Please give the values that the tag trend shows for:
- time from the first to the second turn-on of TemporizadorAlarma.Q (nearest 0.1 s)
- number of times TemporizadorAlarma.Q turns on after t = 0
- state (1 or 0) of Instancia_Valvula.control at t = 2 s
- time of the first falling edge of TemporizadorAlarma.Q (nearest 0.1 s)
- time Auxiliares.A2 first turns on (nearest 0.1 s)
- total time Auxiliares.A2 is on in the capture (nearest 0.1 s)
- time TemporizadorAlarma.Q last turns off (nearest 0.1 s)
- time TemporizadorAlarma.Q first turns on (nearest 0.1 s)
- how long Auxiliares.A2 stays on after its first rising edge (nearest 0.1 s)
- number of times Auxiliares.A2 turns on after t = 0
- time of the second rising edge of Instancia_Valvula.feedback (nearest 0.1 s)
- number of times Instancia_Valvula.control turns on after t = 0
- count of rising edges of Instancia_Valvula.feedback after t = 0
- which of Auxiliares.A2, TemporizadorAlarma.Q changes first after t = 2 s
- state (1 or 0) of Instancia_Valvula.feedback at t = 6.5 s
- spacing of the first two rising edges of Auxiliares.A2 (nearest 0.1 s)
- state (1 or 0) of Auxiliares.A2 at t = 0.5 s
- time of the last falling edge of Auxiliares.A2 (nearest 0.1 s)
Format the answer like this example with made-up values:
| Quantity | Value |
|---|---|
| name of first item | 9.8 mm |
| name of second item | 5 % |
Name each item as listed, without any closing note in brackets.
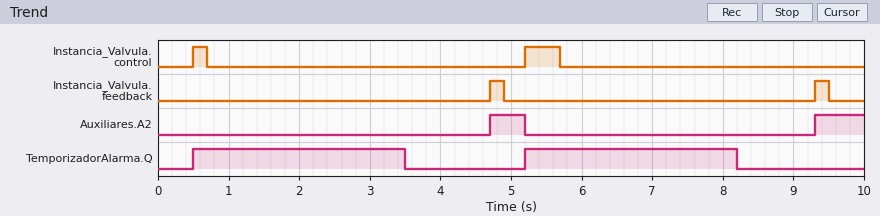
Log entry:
| Quantity | Value |
|---|---|
| time from the first to the second turn-on of TemporizadorAlarma.Q | 4.7 s |
| number of times TemporizadorAlarma.Q turns on after t = 0 | 2 |
| state (1 or 0) of Instancia_Valvula.control at t = 2 s | 0 |
| time of the first falling edge of TemporizadorAlarma.Q | 3.5 s |
| time Auxiliares.A2 first turns on | 4.7 s |
| total time Auxiliares.A2 is on in the capture | 1.2 s |
| time TemporizadorAlarma.Q last turns off | 8.2 s |
| time TemporizadorAlarma.Q first turns on | 0.5 s |
| how long Auxiliares.A2 stays on after its first rising edge | 0.5 s |
| number of times Auxiliares.A2 turns on after t = 0 | 2 |
| time of the second rising edge of Instancia_Valvula.feedback | 9.3 s |
| number of times Instancia_Valvula.control turns on after t = 0 | 2 |
| count of rising edges of Instancia_Valvula.feedback after t = 0 | 2 |
| which of Auxiliares.A2, TemporizadorAlarma.Q changes first after t = 2 s | TemporizadorAlarma.Q |
| state (1 or 0) of Instancia_Valvula.feedback at t = 6.5 s | 0 |
| spacing of the first two rising edges of Auxiliares.A2 | 4.6 s |
| state (1 or 0) of Auxiliares.A2 at t = 0.5 s | 0 |
| time of the last falling edge of Auxiliares.A2 | 5.2 s |
